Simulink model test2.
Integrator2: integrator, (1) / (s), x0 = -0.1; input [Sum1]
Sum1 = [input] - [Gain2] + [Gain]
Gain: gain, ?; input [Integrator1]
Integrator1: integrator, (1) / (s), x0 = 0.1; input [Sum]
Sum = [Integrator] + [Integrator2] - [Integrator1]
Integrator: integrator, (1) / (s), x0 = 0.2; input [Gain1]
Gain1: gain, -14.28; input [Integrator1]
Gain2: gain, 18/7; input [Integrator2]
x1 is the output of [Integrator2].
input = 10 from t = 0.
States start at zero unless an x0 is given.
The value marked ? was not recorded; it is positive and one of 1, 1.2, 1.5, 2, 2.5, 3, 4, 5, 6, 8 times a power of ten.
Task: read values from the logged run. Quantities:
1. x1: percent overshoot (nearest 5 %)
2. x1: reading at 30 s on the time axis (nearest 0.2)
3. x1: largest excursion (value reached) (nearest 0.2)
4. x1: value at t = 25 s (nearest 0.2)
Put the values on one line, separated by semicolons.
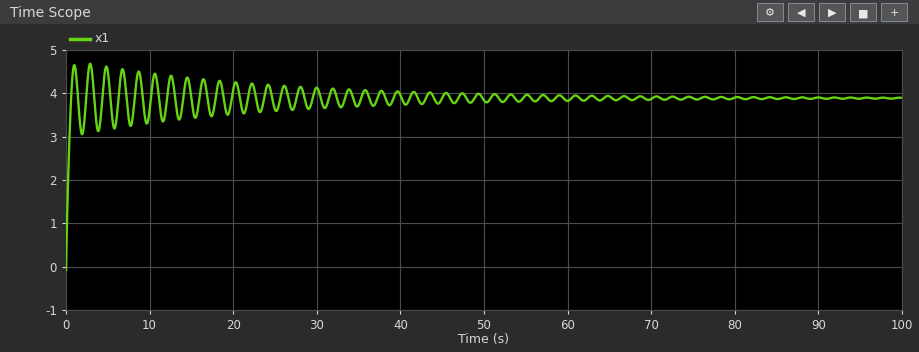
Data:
20 %; 4.2; 4.6; 3.6
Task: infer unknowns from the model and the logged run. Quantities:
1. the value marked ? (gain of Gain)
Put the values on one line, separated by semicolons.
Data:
6
